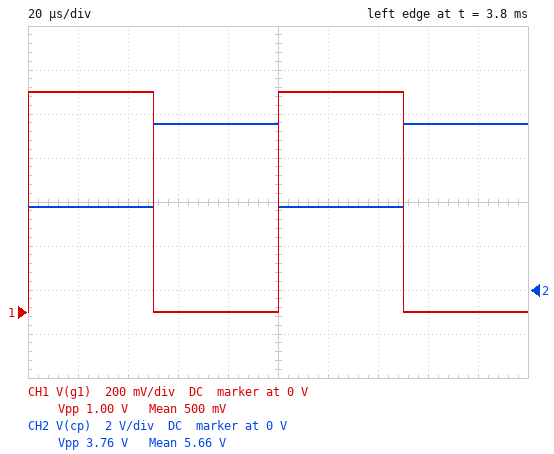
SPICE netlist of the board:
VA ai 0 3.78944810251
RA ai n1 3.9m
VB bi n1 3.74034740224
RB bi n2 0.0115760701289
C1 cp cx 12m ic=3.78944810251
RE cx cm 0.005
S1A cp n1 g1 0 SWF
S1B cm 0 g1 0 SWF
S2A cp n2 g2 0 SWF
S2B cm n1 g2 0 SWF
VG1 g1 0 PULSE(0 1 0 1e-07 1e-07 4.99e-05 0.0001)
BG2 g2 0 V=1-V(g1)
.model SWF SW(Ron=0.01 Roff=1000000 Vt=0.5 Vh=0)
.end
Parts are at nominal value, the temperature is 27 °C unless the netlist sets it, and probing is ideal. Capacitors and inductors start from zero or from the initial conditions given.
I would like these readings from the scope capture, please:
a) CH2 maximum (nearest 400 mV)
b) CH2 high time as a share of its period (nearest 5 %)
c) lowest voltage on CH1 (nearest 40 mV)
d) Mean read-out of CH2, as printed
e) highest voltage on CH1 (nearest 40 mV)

7.6 V
50 %
0 V
5.66 V
1.00 V
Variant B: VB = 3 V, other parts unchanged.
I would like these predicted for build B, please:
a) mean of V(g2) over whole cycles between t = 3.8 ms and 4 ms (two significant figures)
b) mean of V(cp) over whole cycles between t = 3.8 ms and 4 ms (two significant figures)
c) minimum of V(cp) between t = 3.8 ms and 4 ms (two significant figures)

500 mV
5.3 V
3.6 V
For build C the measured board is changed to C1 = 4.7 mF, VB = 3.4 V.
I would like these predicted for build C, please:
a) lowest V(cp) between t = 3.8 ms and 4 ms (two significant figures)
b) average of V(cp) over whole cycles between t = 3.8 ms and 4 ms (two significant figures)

3.7 V
5.5 V
